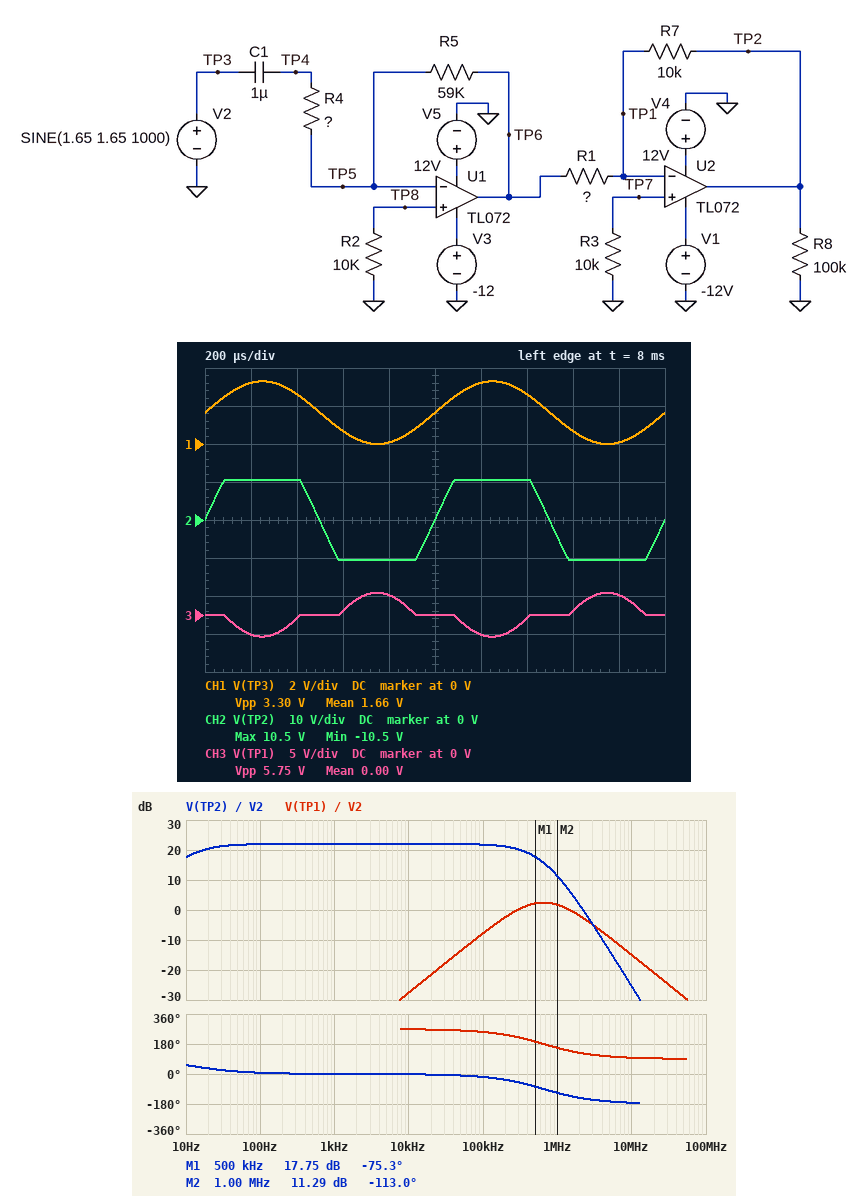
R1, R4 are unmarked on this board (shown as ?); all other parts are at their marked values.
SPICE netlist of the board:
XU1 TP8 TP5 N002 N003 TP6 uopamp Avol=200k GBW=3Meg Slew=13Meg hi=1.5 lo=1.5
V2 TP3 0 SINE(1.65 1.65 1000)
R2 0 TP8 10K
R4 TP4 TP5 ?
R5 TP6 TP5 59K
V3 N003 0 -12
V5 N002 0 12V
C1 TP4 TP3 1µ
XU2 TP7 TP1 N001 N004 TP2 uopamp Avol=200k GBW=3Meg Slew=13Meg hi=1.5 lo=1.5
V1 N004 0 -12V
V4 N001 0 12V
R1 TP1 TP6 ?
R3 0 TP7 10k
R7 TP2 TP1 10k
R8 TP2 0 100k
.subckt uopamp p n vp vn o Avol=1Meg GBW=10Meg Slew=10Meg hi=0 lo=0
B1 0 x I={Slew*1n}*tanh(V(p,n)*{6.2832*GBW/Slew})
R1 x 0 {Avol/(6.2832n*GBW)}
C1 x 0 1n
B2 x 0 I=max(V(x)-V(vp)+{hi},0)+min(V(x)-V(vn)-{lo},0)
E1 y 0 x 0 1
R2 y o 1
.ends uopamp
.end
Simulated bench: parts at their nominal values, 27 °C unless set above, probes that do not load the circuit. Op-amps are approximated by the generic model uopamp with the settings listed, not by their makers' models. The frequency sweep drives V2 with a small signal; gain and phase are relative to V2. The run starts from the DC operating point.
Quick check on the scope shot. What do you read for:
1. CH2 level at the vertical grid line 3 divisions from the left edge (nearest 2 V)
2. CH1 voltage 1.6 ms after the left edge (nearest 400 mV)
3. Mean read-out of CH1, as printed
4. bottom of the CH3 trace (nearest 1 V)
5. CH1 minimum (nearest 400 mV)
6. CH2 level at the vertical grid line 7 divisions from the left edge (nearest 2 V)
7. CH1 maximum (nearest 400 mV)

-10 V
800 mV
1.66 V
-3 V
0 V
10 V
3.2 V
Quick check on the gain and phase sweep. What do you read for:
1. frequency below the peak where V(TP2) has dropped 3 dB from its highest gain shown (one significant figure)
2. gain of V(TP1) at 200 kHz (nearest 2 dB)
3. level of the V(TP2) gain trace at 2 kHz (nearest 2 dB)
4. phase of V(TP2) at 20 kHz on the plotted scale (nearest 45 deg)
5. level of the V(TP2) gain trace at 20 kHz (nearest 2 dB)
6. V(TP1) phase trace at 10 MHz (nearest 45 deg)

10 Hz
-2 dB
22 dB
0 deg
22 dB
90 deg
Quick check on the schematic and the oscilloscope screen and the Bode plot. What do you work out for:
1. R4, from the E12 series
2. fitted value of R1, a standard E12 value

12 kΩ
3.9 kΩ
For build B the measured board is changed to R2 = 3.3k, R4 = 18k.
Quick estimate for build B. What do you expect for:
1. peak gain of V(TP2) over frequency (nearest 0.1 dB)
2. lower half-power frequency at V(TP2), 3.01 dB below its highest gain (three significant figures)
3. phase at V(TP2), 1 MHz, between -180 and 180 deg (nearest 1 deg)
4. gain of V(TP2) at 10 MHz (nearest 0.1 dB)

18.5 dB
8.84 Hz
-105 deg
-26.1 dB
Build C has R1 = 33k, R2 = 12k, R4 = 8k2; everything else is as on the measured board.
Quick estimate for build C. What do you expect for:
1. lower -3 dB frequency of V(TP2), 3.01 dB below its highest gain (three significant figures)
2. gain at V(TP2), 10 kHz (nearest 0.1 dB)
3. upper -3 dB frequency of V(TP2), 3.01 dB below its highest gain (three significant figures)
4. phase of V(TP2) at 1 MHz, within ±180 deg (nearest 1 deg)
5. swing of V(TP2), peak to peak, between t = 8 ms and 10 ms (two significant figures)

19.4 Hz
6.8 dB
357 kHz
-93 deg
6.4 V
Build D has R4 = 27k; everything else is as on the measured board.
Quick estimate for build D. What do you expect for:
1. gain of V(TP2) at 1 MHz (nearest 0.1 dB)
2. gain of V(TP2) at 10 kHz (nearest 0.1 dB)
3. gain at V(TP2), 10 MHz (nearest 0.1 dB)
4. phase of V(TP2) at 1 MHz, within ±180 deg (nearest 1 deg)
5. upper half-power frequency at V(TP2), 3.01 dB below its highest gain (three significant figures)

7.9 dB
15.0 dB
-27.1 dB
-97 deg
572 kHz
